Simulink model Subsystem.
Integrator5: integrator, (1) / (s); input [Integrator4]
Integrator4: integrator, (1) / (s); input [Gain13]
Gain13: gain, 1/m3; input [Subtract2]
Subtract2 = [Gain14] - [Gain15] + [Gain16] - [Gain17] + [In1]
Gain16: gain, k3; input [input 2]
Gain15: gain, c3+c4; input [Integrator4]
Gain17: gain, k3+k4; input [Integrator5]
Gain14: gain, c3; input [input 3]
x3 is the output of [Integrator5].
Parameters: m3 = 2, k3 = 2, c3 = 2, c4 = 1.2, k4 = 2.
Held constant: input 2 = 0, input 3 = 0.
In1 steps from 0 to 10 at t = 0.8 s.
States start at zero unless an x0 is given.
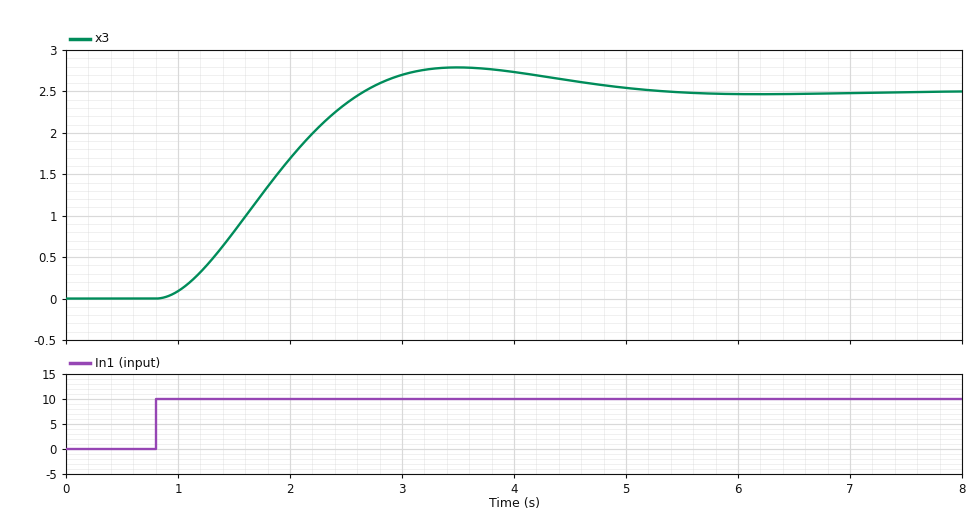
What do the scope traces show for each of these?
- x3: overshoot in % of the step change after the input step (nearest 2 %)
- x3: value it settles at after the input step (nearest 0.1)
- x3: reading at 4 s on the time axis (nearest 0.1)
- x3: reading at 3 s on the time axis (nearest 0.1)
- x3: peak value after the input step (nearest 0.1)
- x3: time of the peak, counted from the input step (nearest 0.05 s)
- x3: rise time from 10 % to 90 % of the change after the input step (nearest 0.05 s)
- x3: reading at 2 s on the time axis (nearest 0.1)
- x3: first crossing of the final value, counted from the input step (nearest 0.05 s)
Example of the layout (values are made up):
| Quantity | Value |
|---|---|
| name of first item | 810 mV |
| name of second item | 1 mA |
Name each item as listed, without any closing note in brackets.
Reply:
| Quantity | Value |
|---|---|
| x3: overshoot in % of the step change after the input step | 12 % |
| x3: value it settles at after the input step | 2.5 |
| x3: reading at 4 s on the time axis | 2.7 |
| x3: reading at 3 s on the time axis | 2.7 |
| x3: peak value after the input step | 2.8 |
| x3: time of the peak, counted from the input step | 2.70 s |
| x3: rise time from 10 % to 90 % of the change after the input step | 1.25 s |
| x3: reading at 2 s on the time axis | 1.7 |
| x3: first crossing of the final value, counted from the input step | 1.85 s |
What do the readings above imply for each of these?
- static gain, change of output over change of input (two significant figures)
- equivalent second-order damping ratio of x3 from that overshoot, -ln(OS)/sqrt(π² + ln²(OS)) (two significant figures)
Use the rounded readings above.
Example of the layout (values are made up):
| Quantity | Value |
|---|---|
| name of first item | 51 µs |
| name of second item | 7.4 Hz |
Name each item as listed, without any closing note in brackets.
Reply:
| Quantity | Value |
|---|---|
| static gain, change of output over change of input | 0.25 |
| equivalent second-order damping ratio of x3 from that overshoot, -ln(OS)/sqrt(π² + ln²(OS)) | 0.56 |
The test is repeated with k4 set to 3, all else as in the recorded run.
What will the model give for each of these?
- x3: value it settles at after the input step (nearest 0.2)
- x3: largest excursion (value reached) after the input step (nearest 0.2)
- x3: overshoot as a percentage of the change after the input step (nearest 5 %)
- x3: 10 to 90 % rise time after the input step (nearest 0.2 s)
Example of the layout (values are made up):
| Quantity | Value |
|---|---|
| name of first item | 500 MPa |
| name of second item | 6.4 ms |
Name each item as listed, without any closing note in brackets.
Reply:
| Quantity | Value |
|---|---|
| x3: value it settles at after the input step | 2.0 |
| x3: largest excursion (value reached) after the input step | 2.4 |
| x3: overshoot as a percentage of the change after the input step | 15 % |
| x3: 10 to 90 % rise time after the input step | 1.0 s |
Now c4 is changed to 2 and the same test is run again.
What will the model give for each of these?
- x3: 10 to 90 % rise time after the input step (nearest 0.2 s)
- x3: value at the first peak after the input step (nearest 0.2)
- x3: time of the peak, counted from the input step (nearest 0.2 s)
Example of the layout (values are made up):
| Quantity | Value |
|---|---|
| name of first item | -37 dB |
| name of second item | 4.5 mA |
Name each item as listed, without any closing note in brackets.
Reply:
| Quantity | Value |
|---|---|
| x3: 10 to 90 % rise time after the input step | 1.6 s |
| x3: value at the first peak after the input step | 2.6 |
| x3: time of the peak, counted from the input step | 3.2 s |
